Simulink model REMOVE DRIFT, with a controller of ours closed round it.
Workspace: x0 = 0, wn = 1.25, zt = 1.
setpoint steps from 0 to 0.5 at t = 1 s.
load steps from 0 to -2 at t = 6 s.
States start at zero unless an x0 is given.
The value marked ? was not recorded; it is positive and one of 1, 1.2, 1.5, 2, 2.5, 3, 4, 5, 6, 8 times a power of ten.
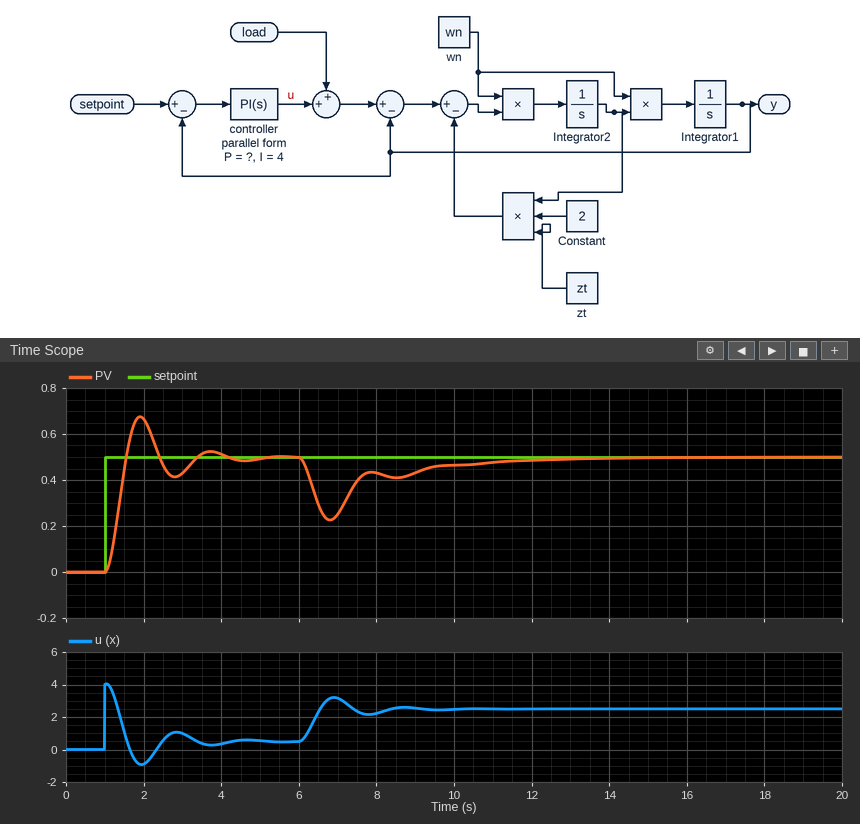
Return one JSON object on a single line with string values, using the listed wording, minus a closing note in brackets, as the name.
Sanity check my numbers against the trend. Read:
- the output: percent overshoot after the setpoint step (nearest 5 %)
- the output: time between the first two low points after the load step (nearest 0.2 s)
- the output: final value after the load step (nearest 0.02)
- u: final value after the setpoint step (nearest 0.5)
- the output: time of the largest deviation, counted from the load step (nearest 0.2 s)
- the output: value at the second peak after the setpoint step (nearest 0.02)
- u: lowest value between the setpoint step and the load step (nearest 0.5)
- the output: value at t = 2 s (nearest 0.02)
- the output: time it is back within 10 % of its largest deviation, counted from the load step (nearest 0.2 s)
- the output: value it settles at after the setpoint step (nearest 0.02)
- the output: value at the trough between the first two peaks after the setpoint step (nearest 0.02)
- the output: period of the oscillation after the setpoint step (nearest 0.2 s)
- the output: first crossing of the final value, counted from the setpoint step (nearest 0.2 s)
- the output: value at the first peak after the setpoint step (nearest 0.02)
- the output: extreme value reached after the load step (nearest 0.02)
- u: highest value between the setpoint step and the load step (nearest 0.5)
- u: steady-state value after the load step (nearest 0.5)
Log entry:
{"the output: percent overshoot after the setpoint step": "35 %", "the output: time between the first two low points after the load step": "1.8 s", "the output: final value after the load step": "0.50", "u: final value after the setpoint step": "0.5", "the output: time of the largest deviation, counted from the load step": "0.8 s", "the output: value at the second peak after the setpoint step": "0.52", "u: lowest value between the setpoint step and the load step": "-1.0", "the output: value at t = 2 s": "0.66", "the output: time it is back within 10 % of its largest deviation, counted from the load step": "4.8 s", "the output: value it settles at after the setpoint step": "0.50", "the output: value at the trough between the first two peaks after the setpoint step": "0.42", "the output: period of the oscillation after the setpoint step": "1.8 s", "the output: first crossing of the final value, counted from the setpoint step": "0.6 s", "the output: value at the first peak after the setpoint step": "0.68", "the output: extreme value reached after the load step": "0.22", "u: highest value between the setpoint step and the load step": "4.0", "u: steady-state value after the load step": "2.5"}
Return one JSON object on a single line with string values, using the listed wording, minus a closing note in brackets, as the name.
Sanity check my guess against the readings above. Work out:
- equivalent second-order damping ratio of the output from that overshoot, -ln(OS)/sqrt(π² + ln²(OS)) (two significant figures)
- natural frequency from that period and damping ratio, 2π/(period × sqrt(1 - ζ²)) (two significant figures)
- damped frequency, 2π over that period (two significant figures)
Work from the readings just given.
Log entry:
{"equivalent second-order damping ratio of the output from that overshoot, -ln(OS)/sqrt(π² + ln²(OS))": "0.32", "natural frequency from that period and damping ratio, 2π/(period × sqrt(1 - ζ²))": "3.7 rad/s", "damped frequency, 2π over that period": "3.5 rad/s"}
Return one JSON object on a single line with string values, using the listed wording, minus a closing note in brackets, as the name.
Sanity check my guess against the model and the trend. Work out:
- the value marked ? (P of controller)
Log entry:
{"the value marked ?": "8"}
